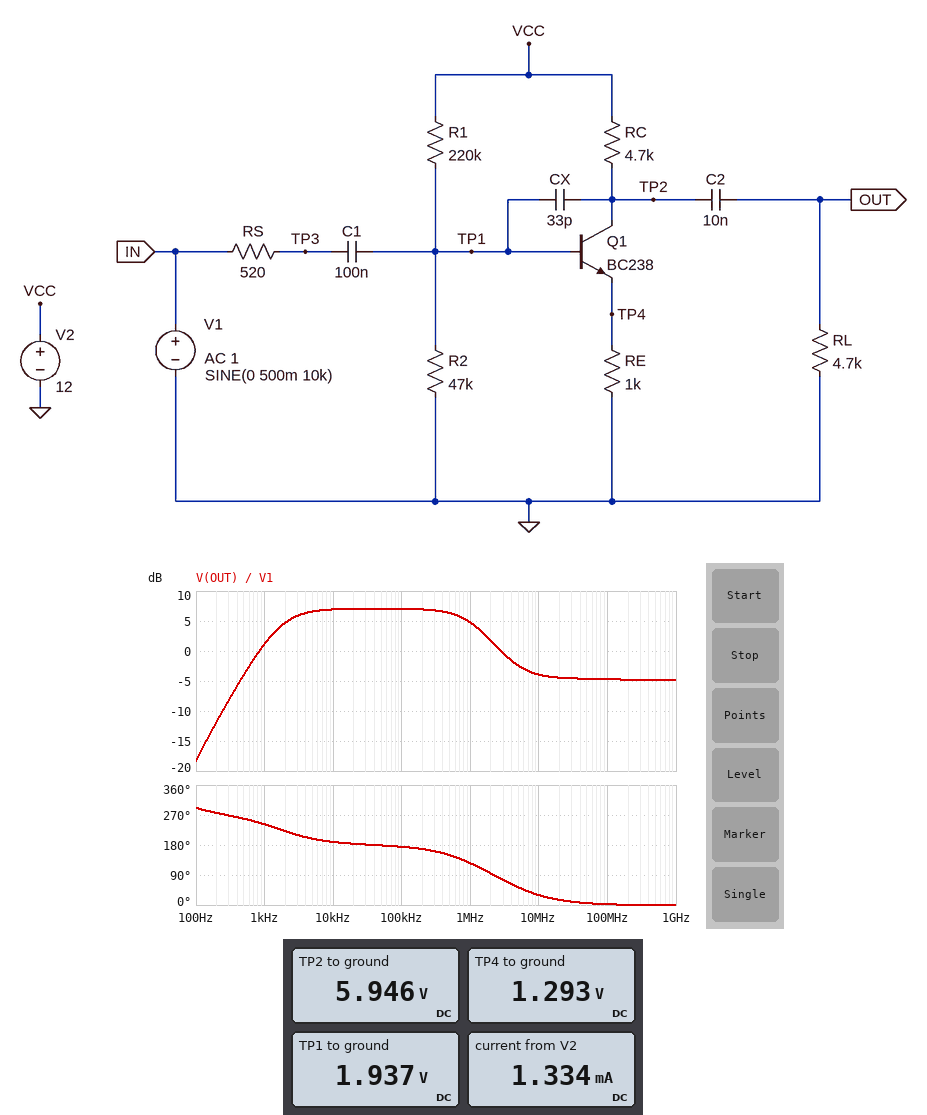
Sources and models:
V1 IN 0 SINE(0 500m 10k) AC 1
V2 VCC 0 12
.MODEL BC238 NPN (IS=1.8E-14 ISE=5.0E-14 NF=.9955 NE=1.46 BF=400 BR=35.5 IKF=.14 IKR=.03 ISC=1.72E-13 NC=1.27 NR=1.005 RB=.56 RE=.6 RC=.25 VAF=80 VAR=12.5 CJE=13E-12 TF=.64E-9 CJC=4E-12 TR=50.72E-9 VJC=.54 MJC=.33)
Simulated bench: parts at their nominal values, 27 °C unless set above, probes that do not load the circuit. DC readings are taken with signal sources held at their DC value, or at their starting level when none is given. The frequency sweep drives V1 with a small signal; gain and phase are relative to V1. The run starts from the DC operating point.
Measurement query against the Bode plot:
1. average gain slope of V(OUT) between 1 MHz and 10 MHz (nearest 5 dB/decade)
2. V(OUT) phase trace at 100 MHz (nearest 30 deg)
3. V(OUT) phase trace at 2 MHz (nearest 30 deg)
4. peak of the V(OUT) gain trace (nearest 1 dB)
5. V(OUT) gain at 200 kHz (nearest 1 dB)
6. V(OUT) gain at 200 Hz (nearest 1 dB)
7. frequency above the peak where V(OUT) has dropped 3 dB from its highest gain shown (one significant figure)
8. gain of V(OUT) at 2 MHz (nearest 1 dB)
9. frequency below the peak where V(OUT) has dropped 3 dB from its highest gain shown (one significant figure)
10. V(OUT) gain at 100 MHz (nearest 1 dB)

-10 dB/decade
0 deg
90 deg
7 dB
7 dB
-12 dB
1 MHz
2 dB
2 kHz
-5 dB
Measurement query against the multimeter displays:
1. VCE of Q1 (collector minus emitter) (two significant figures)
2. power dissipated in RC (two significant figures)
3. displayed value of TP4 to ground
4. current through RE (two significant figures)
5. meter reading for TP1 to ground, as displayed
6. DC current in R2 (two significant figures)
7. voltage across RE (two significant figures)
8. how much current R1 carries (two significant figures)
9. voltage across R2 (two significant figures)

4.7 V
7.8 mW
1.293 V
1.3 mA
1.937 V
41 µA
1.3 V
46 µA
1.9 V
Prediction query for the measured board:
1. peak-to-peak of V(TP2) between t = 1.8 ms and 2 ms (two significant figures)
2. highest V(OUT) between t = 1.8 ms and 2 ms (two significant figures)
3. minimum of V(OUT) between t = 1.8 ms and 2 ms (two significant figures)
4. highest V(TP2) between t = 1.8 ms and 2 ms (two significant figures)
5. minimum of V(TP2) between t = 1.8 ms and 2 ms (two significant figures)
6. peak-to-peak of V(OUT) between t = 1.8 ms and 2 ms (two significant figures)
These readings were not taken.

2.3 V
1.1 V
-1.1 V
7.1 V
4.8 V
2.2 V
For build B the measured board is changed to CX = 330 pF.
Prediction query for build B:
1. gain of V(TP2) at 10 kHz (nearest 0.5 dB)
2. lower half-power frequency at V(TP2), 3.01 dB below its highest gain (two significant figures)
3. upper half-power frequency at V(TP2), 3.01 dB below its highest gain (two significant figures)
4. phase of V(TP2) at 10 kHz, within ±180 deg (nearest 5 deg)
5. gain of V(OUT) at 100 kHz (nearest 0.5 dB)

7.0 dB
43 Hz
2.5 kHz
165 deg
5.0 dB
